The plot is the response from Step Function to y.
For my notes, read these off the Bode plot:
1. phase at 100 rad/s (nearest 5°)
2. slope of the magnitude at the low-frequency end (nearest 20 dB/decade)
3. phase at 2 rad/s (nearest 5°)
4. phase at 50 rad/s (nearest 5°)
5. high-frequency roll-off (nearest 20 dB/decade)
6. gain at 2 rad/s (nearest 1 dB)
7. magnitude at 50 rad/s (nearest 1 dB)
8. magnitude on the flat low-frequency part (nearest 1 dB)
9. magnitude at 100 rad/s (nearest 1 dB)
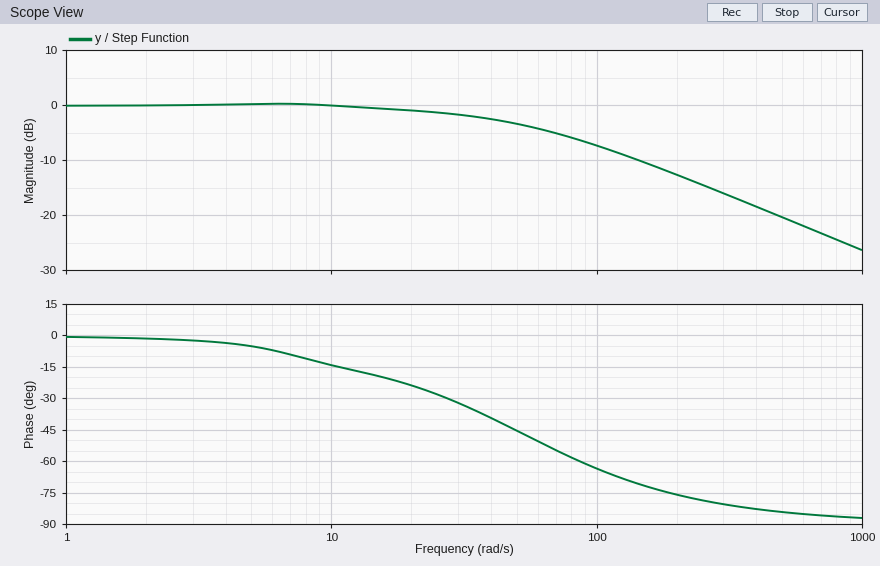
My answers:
-65°
0 dB/decade
0°
-45°
-20 dB/decade
0 dB
-3 dB
0 dB
-7 dB
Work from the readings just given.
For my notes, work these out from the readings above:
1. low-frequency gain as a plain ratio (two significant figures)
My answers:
1.0
